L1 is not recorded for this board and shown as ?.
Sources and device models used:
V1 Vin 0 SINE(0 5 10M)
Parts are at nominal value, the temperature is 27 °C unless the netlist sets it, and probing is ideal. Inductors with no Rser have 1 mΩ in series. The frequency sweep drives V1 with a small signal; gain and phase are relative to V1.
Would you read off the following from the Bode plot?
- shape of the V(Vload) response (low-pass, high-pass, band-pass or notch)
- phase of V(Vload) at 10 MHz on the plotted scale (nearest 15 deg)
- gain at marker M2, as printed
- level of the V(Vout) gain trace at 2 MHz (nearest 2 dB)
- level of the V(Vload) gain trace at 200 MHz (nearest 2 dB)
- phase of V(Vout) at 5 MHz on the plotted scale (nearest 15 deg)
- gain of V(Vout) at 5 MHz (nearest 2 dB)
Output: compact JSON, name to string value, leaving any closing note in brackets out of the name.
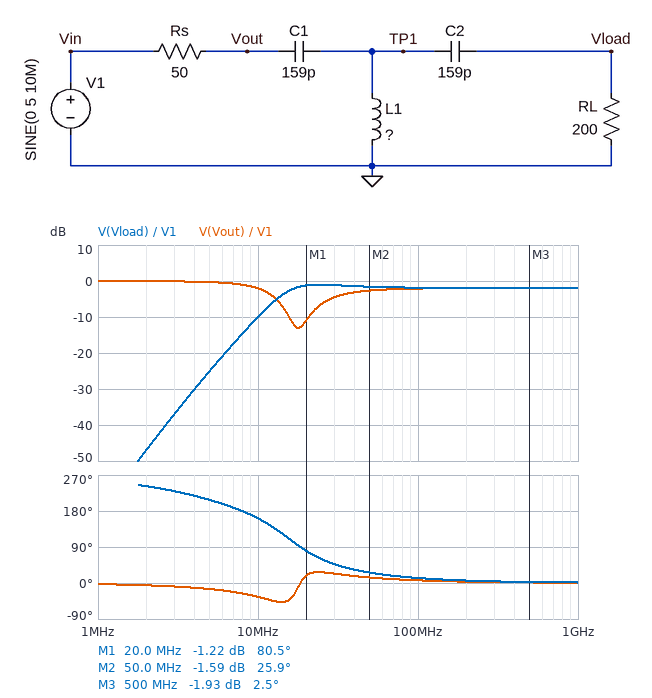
{"shape of the V(Vload) response": "high-pass", "phase of V(Vload) at 10 MHz on the plotted scale": "165 deg", "gain at marker M2, as printed": "-1.59 dB", "level of the V(Vout) gain trace at 2 MHz": "0 dB", "level of the V(Vload) gain trace at 200 MHz": "-2 dB", "phase of V(Vout) at 5 MHz on the plotted scale": "-15 deg", "gain of V(Vout) at 5 MHz": "0 dB"}
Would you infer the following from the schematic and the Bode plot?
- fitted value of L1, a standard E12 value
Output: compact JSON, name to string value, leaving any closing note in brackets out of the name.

{"fitted value of L1, a standard E12 value": "470 nH"}
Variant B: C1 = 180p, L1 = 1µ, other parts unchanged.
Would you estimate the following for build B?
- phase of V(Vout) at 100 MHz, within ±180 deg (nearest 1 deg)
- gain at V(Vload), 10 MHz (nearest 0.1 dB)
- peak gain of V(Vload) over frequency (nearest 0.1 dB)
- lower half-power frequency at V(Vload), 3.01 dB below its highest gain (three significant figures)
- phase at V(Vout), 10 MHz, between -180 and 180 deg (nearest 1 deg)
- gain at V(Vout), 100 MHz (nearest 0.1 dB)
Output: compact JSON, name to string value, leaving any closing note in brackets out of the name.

{"phase of V(Vout) at 100 MHz, within ±180 deg": "3 deg", "gain at V(Vload), 10 MHz": "-1.4 dB", "peak gain of V(Vload) over frequency": "-0.3 dB", "lower half-power frequency at V(Vload), 3.01 dB below its highest gain": "8.72 MHz", "phase at V(Vout), 10 MHz, between -180 and 180 deg": "-31 deg", "gain at V(Vout), 100 MHz": "-2.0 dB"}
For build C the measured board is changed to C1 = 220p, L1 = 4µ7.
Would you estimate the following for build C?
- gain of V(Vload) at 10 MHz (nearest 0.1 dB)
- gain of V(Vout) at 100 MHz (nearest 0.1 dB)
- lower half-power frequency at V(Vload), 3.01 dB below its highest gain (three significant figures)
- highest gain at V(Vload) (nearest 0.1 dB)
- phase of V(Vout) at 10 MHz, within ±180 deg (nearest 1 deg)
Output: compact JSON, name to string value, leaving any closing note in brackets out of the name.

{"gain of V(Vload) at 10 MHz": "-2.2 dB", "gain of V(Vout) at 100 MHz": "-1.9 dB", "lower half-power frequency at V(Vload), 3.01 dB below its highest gain": "3.51 MHz", "highest gain at V(Vload)": "-0.1 dB", "phase of V(Vout) at 10 MHz, within ±180 deg": "0 deg"}
